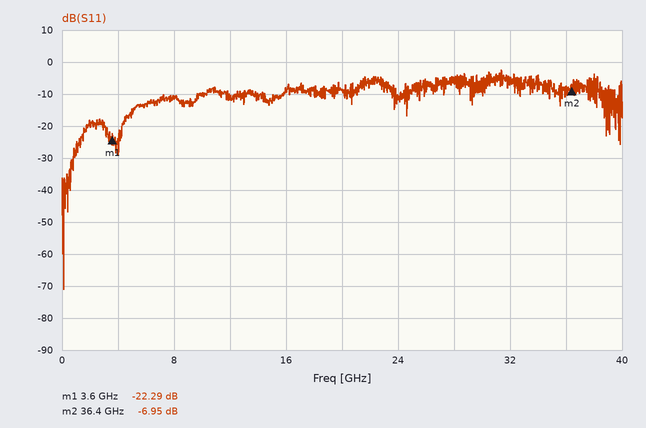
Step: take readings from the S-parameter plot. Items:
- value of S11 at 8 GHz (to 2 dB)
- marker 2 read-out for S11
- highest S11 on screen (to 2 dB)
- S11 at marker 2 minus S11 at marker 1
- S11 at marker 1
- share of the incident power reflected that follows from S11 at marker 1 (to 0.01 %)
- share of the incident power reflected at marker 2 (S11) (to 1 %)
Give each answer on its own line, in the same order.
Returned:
-12 dB
-6.95 dB
-2 dB
15.34 dB
-22.29 dB
0.59 %
20 %
